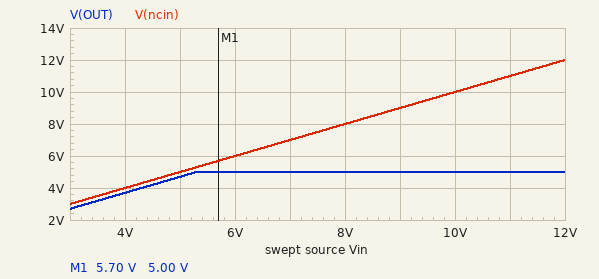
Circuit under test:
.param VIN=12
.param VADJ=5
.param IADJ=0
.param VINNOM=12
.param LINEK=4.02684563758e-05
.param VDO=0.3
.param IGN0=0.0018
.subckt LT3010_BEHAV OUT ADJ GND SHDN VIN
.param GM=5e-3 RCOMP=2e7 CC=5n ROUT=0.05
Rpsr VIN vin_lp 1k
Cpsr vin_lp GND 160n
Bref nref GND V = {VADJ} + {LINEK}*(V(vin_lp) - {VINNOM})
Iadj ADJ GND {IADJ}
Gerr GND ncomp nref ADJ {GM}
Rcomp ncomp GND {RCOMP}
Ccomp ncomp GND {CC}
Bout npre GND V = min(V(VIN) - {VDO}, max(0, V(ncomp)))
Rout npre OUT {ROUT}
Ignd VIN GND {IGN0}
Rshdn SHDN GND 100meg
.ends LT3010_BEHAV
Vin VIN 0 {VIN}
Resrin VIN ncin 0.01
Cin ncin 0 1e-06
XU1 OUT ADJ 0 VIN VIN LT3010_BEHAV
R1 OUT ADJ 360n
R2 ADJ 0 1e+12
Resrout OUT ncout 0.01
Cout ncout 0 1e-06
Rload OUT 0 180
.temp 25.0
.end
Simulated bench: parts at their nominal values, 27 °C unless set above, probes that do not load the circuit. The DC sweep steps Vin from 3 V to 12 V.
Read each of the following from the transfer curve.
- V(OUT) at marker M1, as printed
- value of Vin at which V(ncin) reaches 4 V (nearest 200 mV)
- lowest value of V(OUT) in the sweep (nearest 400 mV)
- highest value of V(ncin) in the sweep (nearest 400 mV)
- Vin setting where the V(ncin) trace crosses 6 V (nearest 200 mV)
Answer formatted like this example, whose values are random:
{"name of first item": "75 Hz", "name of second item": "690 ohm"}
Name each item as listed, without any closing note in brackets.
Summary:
{"V(OUT) at marker M1, as printed": "5.00 V", "value of Vin at which V(ncin) reaches 4 V": "4.0 V", "lowest value of V(OUT) in the sweep": "2.8 V", "highest value of V(ncin) in the sweep": "12.0 V", "Vin setting where the V(ncin) trace crosses 6 V": "6.0 V"}
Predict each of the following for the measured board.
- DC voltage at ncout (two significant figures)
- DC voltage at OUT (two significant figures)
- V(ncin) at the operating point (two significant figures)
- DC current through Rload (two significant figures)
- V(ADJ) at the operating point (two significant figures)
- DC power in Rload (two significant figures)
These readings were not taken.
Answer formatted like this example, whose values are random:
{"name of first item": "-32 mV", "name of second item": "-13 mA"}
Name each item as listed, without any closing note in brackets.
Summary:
{"DC voltage at ncout": "5.0 V", "DC voltage at OUT": "5.0 V", "V(ncin) at the operating point": "12 V", "DC current through Rload": "28 mA", "V(ADJ) at the operating point": "5.0 V", "DC power in Rload": "140 mW"}
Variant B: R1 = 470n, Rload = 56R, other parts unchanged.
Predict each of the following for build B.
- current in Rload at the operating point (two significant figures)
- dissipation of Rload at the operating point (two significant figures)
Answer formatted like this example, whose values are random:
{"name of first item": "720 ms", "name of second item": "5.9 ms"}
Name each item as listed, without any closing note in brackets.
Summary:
{"current in Rload at the operating point": "89 mA", "dissipation of Rload at the operating point": "450 mW"}
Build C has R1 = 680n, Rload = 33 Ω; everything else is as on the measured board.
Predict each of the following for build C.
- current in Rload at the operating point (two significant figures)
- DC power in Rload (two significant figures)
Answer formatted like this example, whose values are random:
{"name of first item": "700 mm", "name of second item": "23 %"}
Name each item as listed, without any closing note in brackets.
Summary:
{"current in Rload at the operating point": "150 mA", "DC power in Rload": "760 mW"}
